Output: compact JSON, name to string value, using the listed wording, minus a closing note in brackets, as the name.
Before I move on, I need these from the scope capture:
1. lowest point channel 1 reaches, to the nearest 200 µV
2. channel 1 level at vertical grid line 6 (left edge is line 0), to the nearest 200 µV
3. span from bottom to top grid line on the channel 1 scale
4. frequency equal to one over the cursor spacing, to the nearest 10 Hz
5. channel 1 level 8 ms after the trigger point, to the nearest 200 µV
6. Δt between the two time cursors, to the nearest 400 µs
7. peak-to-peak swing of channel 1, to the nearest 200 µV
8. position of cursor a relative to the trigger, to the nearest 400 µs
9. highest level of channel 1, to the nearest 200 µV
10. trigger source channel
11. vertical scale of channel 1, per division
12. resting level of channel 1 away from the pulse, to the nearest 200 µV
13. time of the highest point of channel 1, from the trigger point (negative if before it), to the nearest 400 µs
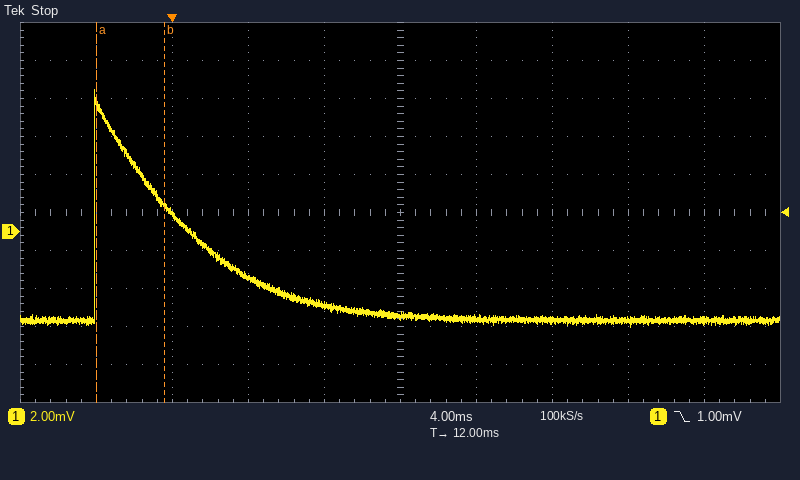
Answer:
{"lowest point channel 1 reaches, to the nearest 200 µV": "-5.0 mV", "channel 1 level at vertical grid line 6 (left edge is line 0), to the nearest 200 µV": "-4.6 mV", "span from bottom to top grid line on the channel 1 scale": "20 mV", "frequency equal to one over the cursor spacing, to the nearest 10 Hz": "280 Hz", "channel 1 level 8 ms after the trigger point, to the nearest 200 µV": "-3.8 mV", "Δt between the two time cursors, to the nearest 400 µs": "3.6 ms", "peak-to-peak swing of channel 1, to the nearest 200 µV": "12.4 mV", "position of cursor a relative to the trigger, to the nearest 400 µs": "-4.0 ms", "highest level of channel 1, to the nearest 200 µV": "7.4 mV", "trigger source channel": "channel 1", "vertical scale of channel 1, per division": "2 mV", "resting level of channel 1 away from the pulse, to the nearest 200 µV": "-4.6 mV", "time of the highest point of channel 1, from the trigger point (negative if before it), to the nearest 400 µs": "-4.0 ms"}
